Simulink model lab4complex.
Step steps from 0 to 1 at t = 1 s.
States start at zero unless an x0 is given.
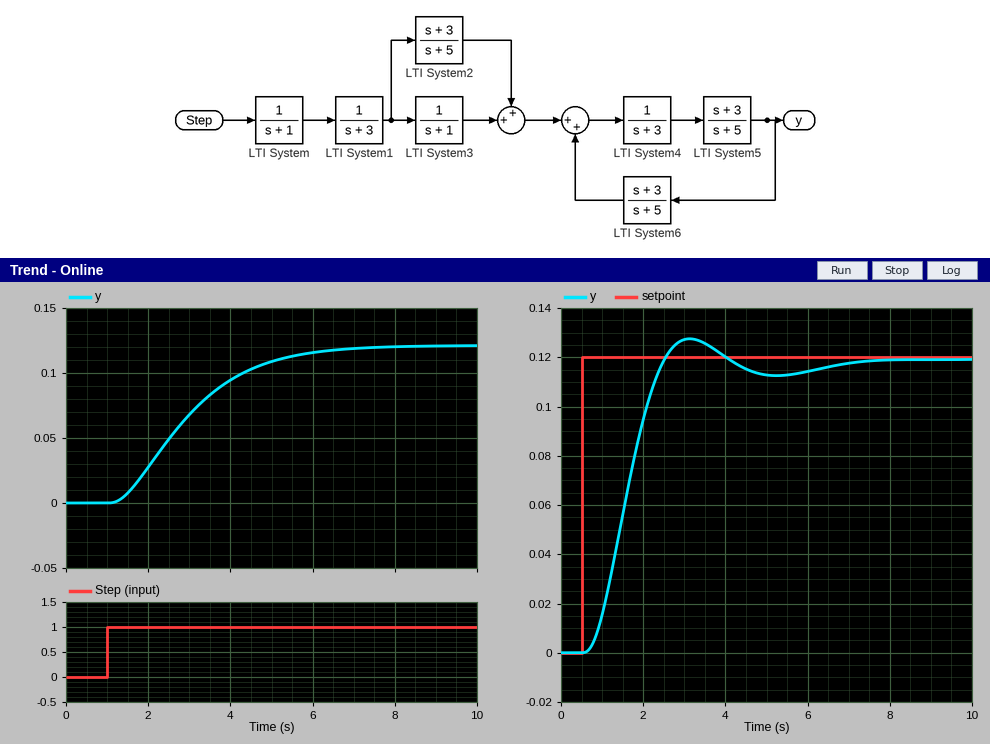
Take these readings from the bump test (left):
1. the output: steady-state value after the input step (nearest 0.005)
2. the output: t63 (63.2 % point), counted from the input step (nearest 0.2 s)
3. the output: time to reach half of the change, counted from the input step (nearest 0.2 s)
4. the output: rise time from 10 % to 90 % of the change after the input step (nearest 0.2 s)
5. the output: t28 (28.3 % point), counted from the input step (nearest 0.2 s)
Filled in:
0.120
2.2 s
1.8 s
3.4 s
1.2 s
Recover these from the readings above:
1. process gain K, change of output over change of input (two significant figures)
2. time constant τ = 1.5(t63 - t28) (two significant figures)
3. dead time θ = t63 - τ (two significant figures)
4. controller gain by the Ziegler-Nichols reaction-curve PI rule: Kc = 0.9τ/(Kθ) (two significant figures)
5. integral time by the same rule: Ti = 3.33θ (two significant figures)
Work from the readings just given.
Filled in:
0.12
1.5 s
0.70 s
16
2.3 s
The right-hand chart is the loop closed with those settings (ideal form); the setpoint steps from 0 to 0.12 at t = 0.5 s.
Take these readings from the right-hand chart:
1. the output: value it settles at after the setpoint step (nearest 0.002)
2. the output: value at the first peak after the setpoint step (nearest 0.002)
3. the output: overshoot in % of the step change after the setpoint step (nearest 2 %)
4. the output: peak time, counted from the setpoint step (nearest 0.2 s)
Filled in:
0.120
0.128
6 %
2.6 s
